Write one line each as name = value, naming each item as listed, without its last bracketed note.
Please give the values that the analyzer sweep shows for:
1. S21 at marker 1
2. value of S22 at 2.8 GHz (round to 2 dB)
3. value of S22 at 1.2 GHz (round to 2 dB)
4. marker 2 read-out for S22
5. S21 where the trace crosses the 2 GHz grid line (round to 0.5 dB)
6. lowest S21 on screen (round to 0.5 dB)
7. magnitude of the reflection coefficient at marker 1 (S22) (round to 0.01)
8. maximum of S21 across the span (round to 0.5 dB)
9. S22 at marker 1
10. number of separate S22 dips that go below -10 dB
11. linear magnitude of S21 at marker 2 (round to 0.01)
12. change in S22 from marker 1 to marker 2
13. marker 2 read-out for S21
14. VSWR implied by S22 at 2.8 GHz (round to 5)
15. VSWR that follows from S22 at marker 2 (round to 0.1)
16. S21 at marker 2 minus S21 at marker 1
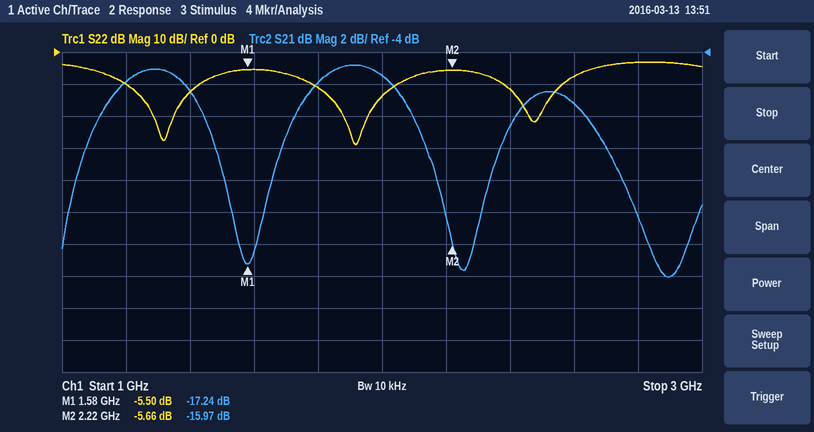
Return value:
S21 at marker 1 = -17.24 dB
value of S22 at 2.8 GHz = -4 dB
value of S22 at 1.2 GHz = -10 dB
marker 2 read-out for S22 = -5.66 dB
S21 where the trace crosses the 2 GHz grid line = -5.5 dB
lowest S21 on screen = -18.0 dB
magnitude of the reflection coefficient at marker 1 (S22) = 0.53
maximum of S21 across the span = -5.0 dB
S22 at marker 1 = -5.50 dB
number of separate S22 dips that go below -10 dB = 3
linear magnitude of S21 at marker 2 = 0.16
change in S22 from marker 1 to marker 2 = -0.16 dB
marker 2 read-out for S21 = -15.97 dB
VSWR implied by S22 at 2.8 GHz = 5
VSWR that follows from S22 at marker 2 = 3.2
S21 at marker 2 minus S21 at marker 1 = 1.27 dB
